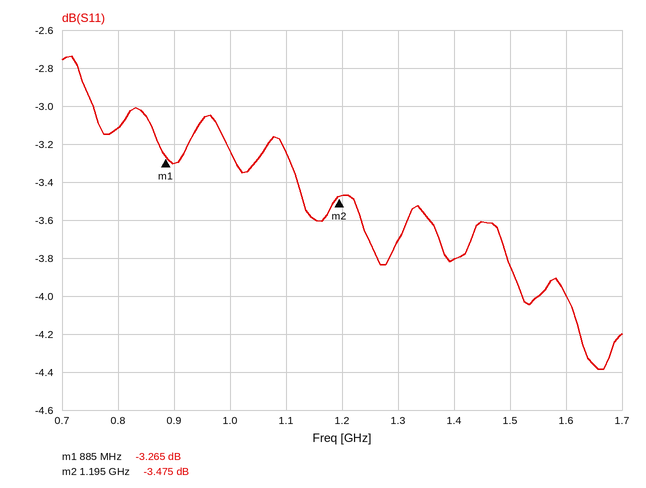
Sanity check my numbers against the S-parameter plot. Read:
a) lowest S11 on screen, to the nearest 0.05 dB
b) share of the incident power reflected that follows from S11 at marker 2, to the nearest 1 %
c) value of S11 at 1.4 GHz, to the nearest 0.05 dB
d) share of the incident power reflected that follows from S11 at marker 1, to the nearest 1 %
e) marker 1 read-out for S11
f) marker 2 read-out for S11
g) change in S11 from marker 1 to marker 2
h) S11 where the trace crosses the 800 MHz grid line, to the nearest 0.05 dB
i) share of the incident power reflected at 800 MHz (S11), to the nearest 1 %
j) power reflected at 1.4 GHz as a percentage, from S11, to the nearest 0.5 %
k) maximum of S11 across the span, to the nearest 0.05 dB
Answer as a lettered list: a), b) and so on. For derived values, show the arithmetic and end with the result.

a) -4.40 dB
b) 10^(-3.475/10) ≈ 45 %
c) -3.80 dB
d) 10^(-3.265/10) ≈ 47 %
e) -3.265 dB
f) -3.475 dB
g) -3.475 − (-3.265) = -0.210 dB
h) -3.10 dB
i) 10^(-3.1/10) ≈ 49 %
j) 10^(-3.8/10) ≈ 41.7 %, so 41.5 % to the nearest 0.5 %
k) -2.75 dB
